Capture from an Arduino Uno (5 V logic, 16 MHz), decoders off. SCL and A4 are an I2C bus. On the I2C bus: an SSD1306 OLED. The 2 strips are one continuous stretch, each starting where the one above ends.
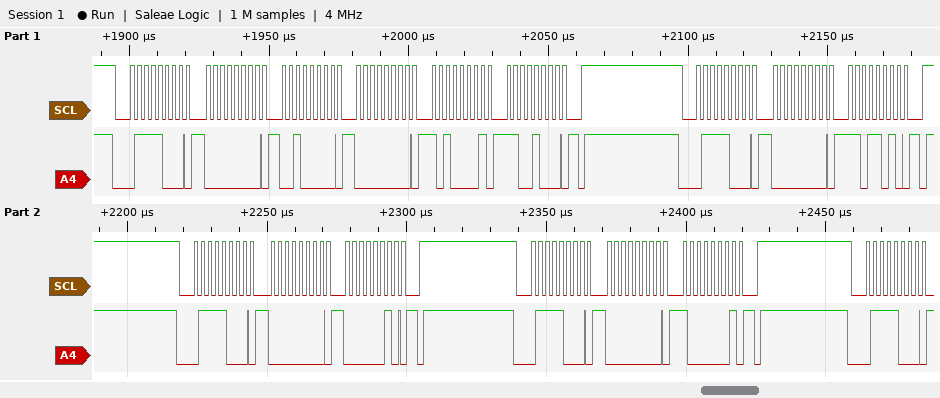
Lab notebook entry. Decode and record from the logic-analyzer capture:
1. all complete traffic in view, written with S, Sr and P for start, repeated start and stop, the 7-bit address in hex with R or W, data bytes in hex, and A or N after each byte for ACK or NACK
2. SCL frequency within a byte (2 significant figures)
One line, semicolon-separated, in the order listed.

S 3CW A 00 A 20 A 00 A A1 A C8 A P S 3CW A 00 A DA A P S 3CW A 00 A 02 A P S 3CW A 00 A 81 A P S 3CW A; 400 kHz
